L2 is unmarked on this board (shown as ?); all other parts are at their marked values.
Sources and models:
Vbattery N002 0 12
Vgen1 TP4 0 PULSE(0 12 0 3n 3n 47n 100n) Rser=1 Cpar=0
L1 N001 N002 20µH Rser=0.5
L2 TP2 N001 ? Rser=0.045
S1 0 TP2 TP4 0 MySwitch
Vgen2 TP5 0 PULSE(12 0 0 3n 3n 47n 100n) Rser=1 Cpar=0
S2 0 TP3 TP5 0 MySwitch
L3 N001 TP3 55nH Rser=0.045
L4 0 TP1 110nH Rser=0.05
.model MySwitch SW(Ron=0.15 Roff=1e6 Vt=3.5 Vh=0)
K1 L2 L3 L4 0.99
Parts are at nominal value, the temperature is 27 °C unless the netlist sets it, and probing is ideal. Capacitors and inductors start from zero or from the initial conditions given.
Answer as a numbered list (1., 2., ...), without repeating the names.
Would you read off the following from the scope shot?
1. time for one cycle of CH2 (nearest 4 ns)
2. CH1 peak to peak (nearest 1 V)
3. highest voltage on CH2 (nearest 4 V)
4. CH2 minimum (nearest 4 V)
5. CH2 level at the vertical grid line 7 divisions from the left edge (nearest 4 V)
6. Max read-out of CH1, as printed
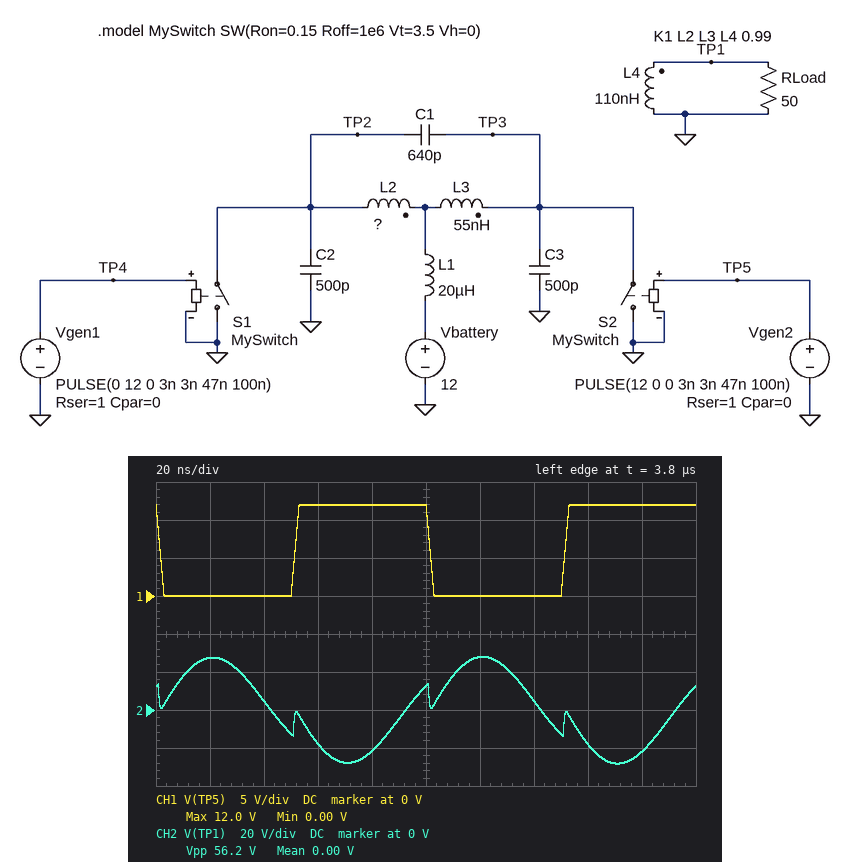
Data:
1. 100 ns
2. 12 V
3. 28 V
4. -28 V
5. 4 V
6. 12.0 V
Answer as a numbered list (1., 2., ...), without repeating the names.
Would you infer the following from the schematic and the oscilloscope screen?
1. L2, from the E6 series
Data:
1. 22 nH
